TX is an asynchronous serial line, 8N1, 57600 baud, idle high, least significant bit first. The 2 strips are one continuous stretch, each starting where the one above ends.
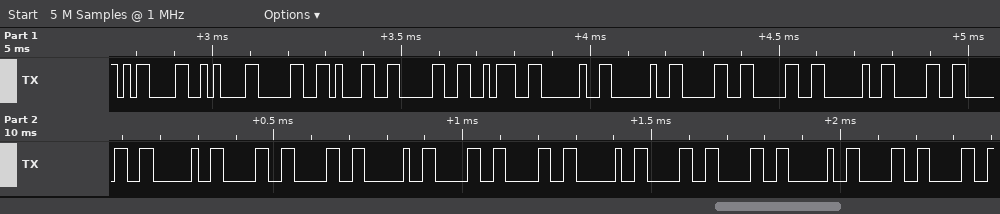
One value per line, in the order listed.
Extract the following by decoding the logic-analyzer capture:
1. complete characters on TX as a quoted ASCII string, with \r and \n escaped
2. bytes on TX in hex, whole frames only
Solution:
"\r\n010:  00 00 00 00 00 00"
0D 0A 30 31 30 3A 20 20 30 30 20 30 30 20 30 30 20 30 30 20 30 30 20 30 30
